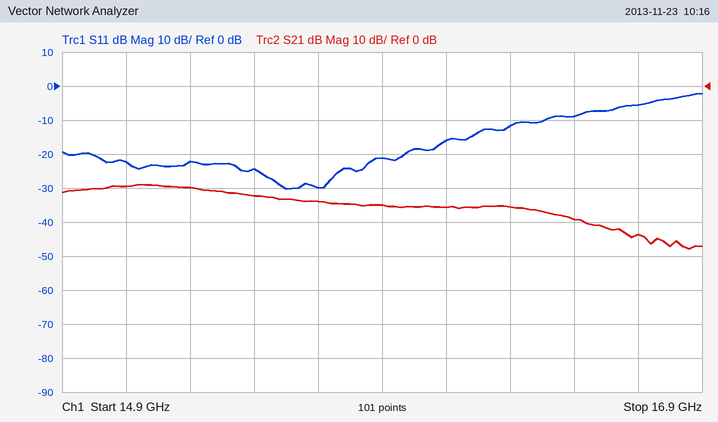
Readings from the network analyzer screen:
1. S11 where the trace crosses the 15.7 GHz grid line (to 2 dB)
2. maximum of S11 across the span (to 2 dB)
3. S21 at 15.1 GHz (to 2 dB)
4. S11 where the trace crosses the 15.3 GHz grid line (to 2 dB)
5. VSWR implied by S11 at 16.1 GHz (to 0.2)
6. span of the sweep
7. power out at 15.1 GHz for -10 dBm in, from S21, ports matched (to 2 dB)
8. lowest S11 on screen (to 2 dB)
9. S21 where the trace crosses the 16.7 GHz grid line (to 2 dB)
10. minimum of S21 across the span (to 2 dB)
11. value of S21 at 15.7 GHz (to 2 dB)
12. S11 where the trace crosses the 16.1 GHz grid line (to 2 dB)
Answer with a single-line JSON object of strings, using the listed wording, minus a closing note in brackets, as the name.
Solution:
{"S11 where the trace crosses the 15.7 GHz grid line": "-30 dB", "maximum of S11 across the span": "-2 dB", "S21 at 15.1 GHz": "-30 dB", "S11 where the trace crosses the 15.3 GHz grid line": "-22 dB", "VSWR implied by S11 at 16.1 GHz": "1.4", "span of the sweep": "2 GHz", "power out at 15.1 GHz for -10 dBm in, from S21, ports matched": "-40 dBm", "lowest S11 on screen": "-30 dB", "S21 where the trace crosses the 16.7 GHz grid line": "-44 dB", "minimum of S21 across the span": "-48 dB", "value of S21 at 15.7 GHz": "-34 dB", "S11 where the trace crosses the 16.1 GHz grid line": "-16 dB"}
